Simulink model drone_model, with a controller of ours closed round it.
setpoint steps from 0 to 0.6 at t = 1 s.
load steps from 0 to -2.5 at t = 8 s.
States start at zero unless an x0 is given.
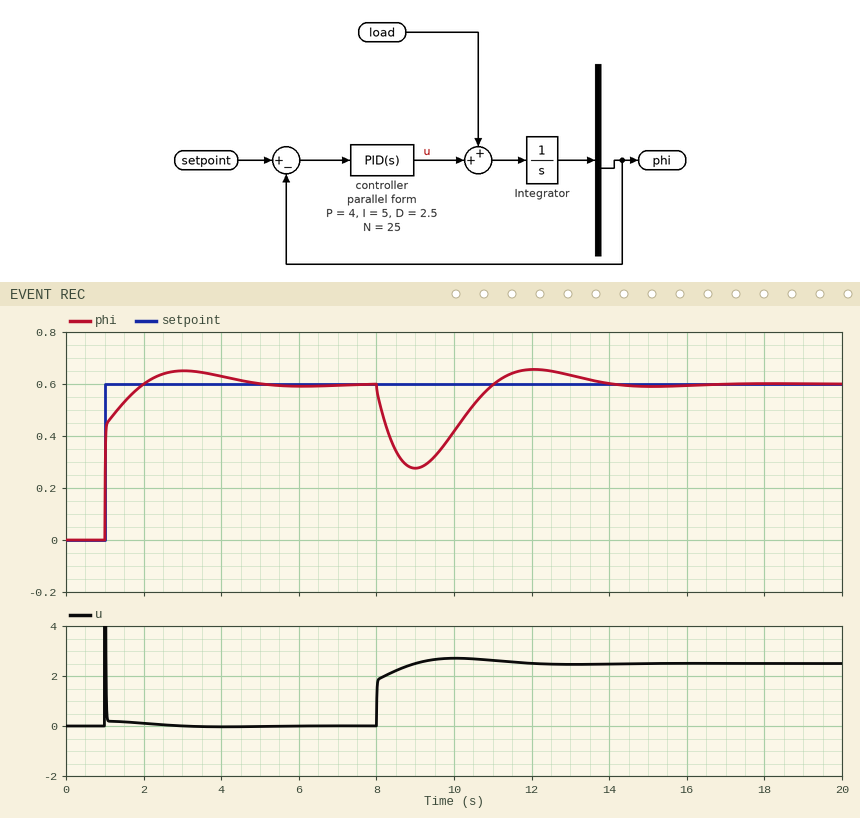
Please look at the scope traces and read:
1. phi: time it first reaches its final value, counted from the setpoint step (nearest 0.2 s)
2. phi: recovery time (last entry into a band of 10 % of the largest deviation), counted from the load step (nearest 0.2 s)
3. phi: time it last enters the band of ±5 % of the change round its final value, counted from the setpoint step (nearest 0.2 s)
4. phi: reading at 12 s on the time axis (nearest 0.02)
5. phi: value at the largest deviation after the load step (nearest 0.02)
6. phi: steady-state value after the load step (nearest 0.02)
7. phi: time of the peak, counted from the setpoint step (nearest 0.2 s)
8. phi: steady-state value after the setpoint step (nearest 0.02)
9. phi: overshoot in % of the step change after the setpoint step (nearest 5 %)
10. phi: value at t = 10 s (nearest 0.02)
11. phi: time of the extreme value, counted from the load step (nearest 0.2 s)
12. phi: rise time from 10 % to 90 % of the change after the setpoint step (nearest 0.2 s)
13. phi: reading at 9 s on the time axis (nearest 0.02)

1.0 s
5.0 s
3.0 s
0.66
0.28
0.60
2.0 s
0.60
10 %
0.42
1.0 s
0.6 s
0.28
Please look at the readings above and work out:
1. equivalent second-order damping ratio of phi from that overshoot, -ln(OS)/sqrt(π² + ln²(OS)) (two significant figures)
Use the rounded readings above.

0.59
